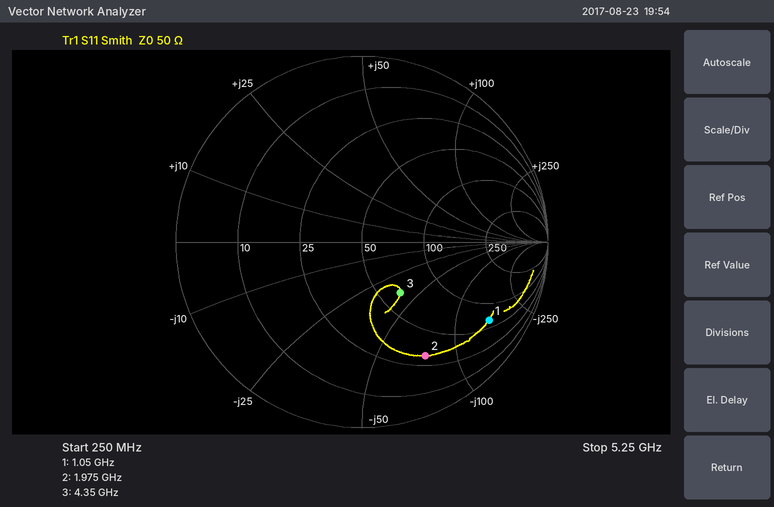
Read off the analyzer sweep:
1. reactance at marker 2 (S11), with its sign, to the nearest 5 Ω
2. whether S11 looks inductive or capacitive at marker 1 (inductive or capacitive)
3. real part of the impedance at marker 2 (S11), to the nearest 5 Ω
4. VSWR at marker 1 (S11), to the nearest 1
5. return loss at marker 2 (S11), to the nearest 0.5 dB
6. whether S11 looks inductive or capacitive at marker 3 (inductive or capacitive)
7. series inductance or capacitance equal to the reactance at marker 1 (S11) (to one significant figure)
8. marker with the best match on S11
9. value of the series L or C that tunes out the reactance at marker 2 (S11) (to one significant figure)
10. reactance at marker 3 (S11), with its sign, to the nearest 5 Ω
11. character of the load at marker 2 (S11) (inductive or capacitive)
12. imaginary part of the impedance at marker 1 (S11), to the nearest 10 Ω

-75 Ω
capacitive
30 Ω
9
3.0 dB
capacitive
1.0 pF
marker 3
6 nH
-40 Ω
capacitive
-150 Ω
